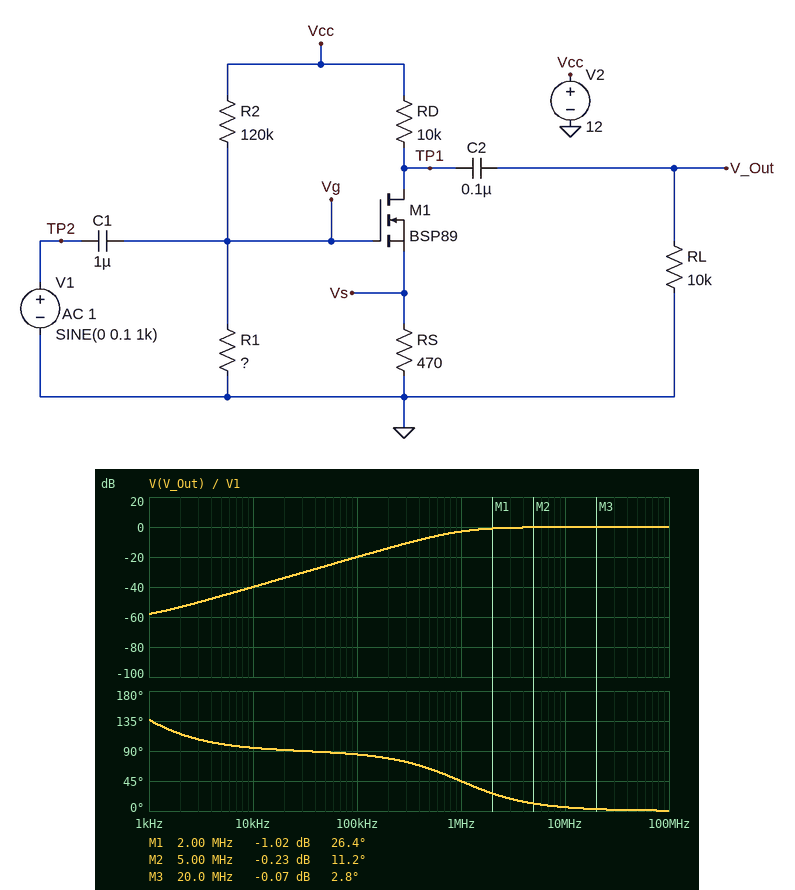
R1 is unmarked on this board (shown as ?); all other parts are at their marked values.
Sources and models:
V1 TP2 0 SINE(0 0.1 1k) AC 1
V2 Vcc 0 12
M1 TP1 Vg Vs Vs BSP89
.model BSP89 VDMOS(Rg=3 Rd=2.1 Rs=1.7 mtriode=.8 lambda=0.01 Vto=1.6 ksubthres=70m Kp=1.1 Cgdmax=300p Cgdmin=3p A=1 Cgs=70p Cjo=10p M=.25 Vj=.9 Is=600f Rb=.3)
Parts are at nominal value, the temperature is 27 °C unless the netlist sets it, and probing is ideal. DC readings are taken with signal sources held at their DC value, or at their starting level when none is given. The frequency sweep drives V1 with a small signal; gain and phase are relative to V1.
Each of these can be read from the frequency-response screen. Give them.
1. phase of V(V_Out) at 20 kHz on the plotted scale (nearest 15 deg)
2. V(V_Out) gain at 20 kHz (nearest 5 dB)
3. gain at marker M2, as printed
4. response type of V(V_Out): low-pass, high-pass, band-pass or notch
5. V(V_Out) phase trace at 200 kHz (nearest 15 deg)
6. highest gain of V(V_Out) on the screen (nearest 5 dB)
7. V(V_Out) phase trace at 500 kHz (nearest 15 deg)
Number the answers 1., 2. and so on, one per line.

1. 90 deg
2. -35 dB
3. -0.23 dB
4. high-pass
5. 75 deg
6. 0 dB
7. 60 deg
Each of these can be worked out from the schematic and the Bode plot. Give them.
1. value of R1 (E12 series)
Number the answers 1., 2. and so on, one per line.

1. 47 kΩ
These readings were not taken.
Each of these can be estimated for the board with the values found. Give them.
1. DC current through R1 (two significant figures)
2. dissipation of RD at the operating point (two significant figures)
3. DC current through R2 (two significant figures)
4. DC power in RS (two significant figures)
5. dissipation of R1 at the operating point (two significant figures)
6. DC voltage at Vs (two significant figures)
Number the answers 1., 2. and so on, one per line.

1. 72 µA
2. 13 mW
3. 72 µA
4. 620 µW
5. 240 µW
6. 540 mV
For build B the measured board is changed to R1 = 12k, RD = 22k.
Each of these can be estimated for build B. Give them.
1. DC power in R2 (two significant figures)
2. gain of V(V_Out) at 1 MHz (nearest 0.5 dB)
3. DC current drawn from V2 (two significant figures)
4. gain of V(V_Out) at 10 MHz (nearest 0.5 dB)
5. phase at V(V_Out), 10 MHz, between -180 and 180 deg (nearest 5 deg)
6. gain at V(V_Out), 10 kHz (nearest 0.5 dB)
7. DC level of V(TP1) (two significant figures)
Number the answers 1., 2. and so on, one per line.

1. 990 µW
2. -6.5 dB
3. 91 µA
4. -0.5 dB
5. 15 deg
6. -44.5 dB
7. 12 V
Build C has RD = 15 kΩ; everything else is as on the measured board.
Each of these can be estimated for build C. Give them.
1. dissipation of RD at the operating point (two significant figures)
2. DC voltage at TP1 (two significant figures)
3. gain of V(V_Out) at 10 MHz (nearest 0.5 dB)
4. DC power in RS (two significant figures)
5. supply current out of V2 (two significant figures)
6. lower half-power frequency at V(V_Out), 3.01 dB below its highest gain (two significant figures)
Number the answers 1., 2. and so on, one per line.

1. 9.0 mW
2. 370 mV
3. 0 dB
4. 280 µW
5. 850 µA
6. 980 kHz
